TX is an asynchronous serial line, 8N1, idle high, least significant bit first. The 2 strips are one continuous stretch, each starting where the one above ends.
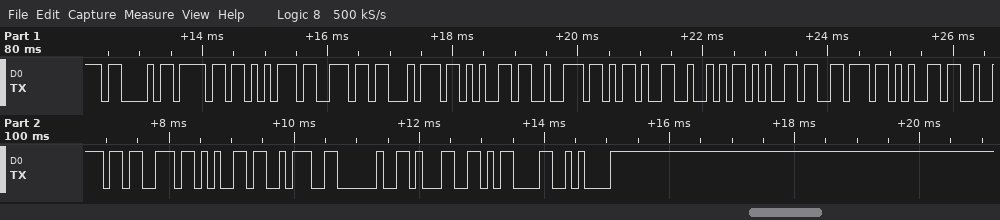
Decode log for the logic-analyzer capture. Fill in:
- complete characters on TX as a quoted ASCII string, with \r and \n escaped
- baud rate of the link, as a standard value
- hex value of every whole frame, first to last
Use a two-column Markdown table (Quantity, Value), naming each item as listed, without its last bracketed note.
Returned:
| Quantity | Value |
|---|---|
| complete characters on TX as a quoted ASCII string, with \r and \n escaped | "Counter-Reverse: 1\r\n" |
| baud rate of the link, as a standard value | 9600 baud |
| hex value of every whole frame, first to last | 43 6F 75 6E 74 65 72 2D 52 65 76 65 72 73 65 3A 20 31 0D 0A |
